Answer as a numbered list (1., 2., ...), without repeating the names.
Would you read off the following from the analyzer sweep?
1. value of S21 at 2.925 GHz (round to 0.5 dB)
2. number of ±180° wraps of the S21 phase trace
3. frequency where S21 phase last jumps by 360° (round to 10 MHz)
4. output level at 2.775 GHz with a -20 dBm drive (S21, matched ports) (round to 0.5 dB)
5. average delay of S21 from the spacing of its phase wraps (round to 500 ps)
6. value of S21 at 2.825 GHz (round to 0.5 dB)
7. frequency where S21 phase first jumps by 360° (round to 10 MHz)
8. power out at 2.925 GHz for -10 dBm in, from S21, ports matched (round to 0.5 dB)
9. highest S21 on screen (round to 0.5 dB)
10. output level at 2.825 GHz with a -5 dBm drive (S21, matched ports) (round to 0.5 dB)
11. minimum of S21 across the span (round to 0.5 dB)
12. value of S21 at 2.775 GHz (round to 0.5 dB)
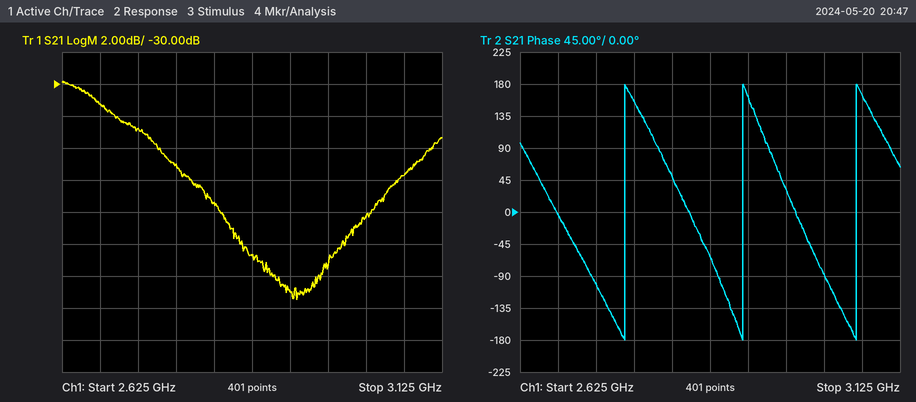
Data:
1. -43.0 dB
2. 3
3. 3.07 GHz
4. -55.0 dBm
5. 6.5 ns
6. -37.5 dB
7. 2.76 GHz
8. -53.0 dBm
9. -30.0 dB
10. -42.5 dBm
11. -43.5 dB
12. -35.0 dB
